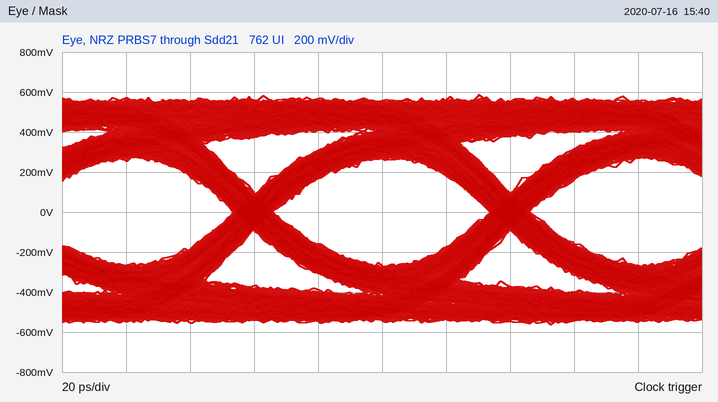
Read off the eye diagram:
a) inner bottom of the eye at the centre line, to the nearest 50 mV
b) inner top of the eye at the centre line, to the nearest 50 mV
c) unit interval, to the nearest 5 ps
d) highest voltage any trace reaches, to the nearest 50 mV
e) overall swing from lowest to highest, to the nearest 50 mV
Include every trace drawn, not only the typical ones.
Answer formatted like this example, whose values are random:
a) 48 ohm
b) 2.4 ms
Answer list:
a) -250 mV
b) 250 mV
c) 80 ps
d) 600 mV
e) 1.15 V
